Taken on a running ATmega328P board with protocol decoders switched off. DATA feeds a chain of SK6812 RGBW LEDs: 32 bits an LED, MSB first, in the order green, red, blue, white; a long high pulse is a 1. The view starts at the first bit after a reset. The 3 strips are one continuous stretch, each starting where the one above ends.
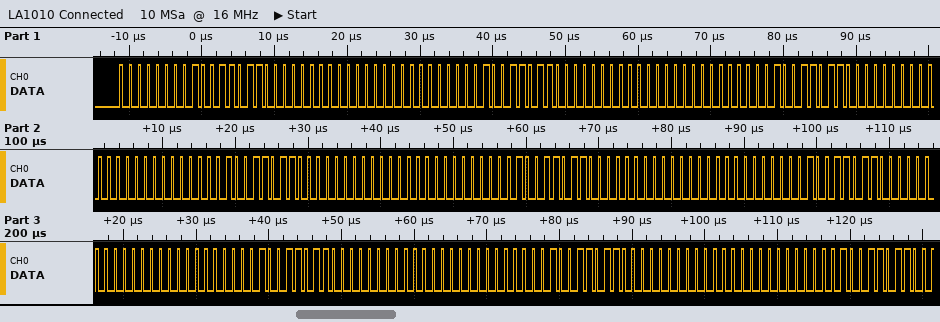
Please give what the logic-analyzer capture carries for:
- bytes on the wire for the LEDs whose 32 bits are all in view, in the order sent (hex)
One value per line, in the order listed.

00 9B 00 00 00 9B 00 00 00 9B 00 00 00 9B 00 00 00 9B 00 00 00 9B 00 00 00 9B 00 00 00 9B 00 00
